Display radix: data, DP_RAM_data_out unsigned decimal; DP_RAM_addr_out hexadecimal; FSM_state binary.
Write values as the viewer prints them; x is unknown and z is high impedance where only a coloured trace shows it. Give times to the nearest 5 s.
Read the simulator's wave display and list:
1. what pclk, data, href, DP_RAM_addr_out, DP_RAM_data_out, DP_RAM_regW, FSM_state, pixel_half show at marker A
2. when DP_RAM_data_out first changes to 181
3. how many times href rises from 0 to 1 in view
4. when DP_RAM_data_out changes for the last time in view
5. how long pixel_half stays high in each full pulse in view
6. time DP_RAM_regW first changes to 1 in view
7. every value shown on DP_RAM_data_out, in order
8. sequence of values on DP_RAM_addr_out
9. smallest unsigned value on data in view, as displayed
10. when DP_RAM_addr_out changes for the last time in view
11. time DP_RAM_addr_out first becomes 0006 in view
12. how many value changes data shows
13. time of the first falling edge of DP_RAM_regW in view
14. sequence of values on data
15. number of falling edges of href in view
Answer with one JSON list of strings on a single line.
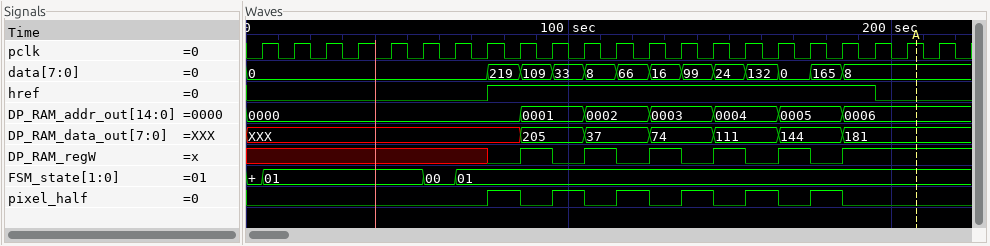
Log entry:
["pclk=1, data=8, href=0, DP_RAM_addr_out=0006, DP_RAM_data_out=181, DP_RAM_regW=1, FSM_state=01, pixel_half=0", "185 s", "1", "185 s", "10 s, 10 s, 10 s, 10 s, 10 s, 10 s", "85 s", "XXX, 205, 37, 74, 111, 144, 181", "0000, 0001, 0002, 0003, 0004, 0005, 0006", "0", "185 s", "185 s", "12", "95 s", "0, 219, 109, 33, 8, 66, 16, 99, 24, 132, 0, 165, 8", "1"]
